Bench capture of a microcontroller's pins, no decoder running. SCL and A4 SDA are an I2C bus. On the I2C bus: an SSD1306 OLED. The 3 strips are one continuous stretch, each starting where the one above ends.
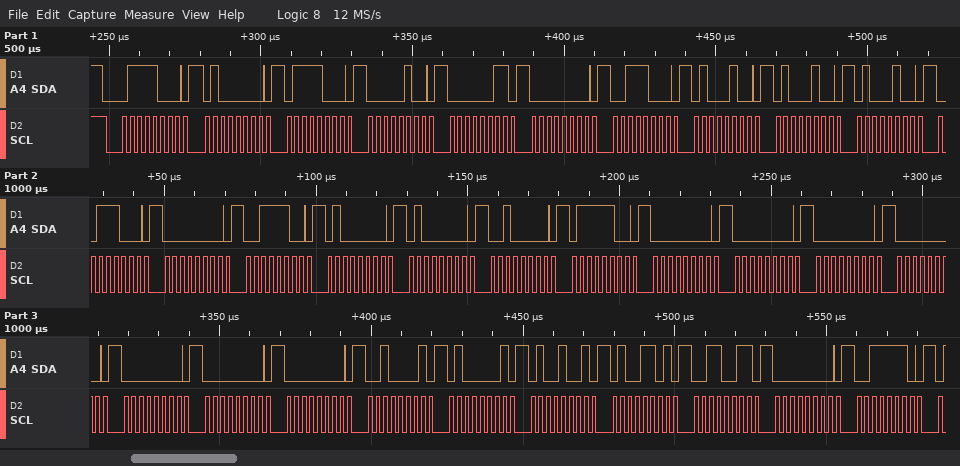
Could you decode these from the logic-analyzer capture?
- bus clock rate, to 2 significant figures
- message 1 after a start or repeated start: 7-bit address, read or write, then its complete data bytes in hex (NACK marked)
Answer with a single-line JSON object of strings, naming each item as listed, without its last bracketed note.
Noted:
{"bus clock rate, to 2 significant figures": "400 kHz", "message 1 after a start or repeated start: 7-bit address, read or write, then its complete data bytes in hex": "0x3C write: 40 78 04 03 00 38 44 44 44 38 00 3C 40 40 20 7C 00 00 00 00 00 00 00 21 41 49 4D 33 00 3E"}
